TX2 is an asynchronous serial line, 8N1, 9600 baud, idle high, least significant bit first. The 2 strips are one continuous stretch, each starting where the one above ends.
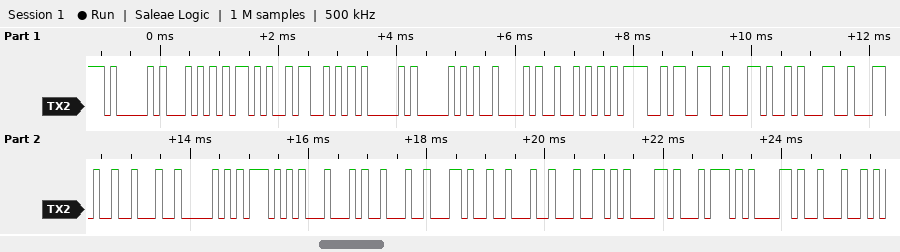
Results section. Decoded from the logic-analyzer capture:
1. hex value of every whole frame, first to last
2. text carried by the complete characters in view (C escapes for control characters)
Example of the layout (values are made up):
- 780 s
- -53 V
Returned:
- 0x41 0x54 0x2B 0x53 0x41 0x50 0x42 0x52 0x3D 0x33 0x2C 0x31 0x2C 0x22 0x50 0x57 0x44 0x22 0x2C 0x22 0x64 0x61 0x74 0x61 0x22
- "AT+SAPBR=3,1,\"PWD\",\"data\""
